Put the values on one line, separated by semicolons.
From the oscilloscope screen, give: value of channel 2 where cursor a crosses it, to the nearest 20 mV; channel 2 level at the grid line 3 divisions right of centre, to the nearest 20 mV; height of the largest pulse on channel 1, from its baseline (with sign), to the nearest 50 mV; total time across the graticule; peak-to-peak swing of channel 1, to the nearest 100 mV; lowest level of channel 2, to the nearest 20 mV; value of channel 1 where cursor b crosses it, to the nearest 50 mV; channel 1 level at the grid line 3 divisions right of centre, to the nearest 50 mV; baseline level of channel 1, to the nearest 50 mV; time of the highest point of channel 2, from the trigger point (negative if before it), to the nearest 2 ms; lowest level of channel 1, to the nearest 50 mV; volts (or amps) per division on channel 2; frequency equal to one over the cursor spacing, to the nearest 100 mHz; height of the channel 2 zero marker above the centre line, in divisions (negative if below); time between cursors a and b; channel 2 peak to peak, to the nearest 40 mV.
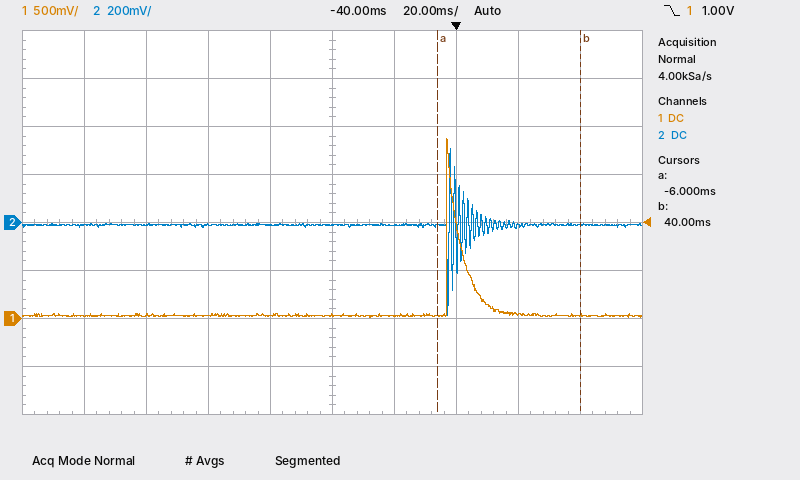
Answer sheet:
-20 mV; -20 mV; +1.85 V; 200 ms; 1.90 V; -380 mV; 50 mV; 50 mV; 50 mV; -2 ms; 0 mV; 200 mV; 21.7 Hz; 0.0 div; 46 ms; 680 mV
